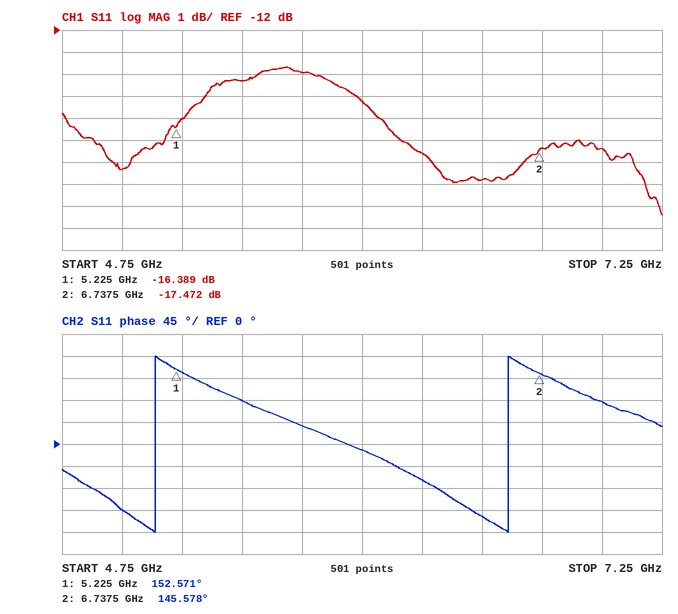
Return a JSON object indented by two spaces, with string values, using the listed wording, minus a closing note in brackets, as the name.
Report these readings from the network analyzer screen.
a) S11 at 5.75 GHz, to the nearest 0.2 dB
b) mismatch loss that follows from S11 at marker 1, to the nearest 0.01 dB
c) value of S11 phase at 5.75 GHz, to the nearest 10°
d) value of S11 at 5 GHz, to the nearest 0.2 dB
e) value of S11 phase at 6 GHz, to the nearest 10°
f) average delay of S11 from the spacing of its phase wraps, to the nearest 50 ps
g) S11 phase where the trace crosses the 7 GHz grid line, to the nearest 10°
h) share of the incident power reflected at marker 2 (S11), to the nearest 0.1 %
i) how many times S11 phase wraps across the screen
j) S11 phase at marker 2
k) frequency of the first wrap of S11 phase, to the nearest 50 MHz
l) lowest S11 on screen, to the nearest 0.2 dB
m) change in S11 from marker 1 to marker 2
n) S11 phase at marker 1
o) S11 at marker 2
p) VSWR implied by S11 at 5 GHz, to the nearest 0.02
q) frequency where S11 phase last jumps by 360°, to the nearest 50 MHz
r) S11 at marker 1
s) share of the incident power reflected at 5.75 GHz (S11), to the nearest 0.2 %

{
  "S11 at 5.75 GHz, to the nearest 0.2 dB": "-14.0 dB",
  "mismatch loss that follows from S11 at marker 1, to the nearest 0.01 dB": "0.10 dB",
  "value of S11 phase at 5.75 GHz, to the nearest 10°": "40°",
  "value of S11 at 5 GHz, to the nearest 0.2 dB": "-18.4 dB",
  "value of S11 phase at 6 GHz, to the nearest 10°": "-10°",
  "average delay of S11 from the spacing of its phase wraps, to the nearest 50 ps": "700 ps",
  "S11 phase where the trace crosses the 7 GHz grid line, to the nearest 10°": "90°",
  "share of the incident power reflected at marker 2 (S11), to the nearest 0.1 %": "1.8 %",
  "how many times S11 phase wraps across the screen": "2",
  "S11 phase at marker 2": "145.578°",
  "frequency of the first wrap of S11 phase, to the nearest 50 MHz": "5.15 GHz",
  "lowest S11 on screen, to the nearest 0.2 dB": "-20.4 dB",
  "change in S11 from marker 1 to marker 2": "-1.083 dB",
  "S11 phase at marker 1": "152.571°",
  "S11 at marker 2": "-17.472 dB",
  "VSWR implied by S11 at 5 GHz, to the nearest 0.02": "1.28",
  "frequency where S11 phase last jumps by 360°, to the nearest 50 MHz": "6.60 GHz",
  "S11 at marker 1": "-16.389 dB",
  "share of the incident power reflected at 5.75 GHz (S11), to the nearest 0.2 %": "4.0 %"
}
